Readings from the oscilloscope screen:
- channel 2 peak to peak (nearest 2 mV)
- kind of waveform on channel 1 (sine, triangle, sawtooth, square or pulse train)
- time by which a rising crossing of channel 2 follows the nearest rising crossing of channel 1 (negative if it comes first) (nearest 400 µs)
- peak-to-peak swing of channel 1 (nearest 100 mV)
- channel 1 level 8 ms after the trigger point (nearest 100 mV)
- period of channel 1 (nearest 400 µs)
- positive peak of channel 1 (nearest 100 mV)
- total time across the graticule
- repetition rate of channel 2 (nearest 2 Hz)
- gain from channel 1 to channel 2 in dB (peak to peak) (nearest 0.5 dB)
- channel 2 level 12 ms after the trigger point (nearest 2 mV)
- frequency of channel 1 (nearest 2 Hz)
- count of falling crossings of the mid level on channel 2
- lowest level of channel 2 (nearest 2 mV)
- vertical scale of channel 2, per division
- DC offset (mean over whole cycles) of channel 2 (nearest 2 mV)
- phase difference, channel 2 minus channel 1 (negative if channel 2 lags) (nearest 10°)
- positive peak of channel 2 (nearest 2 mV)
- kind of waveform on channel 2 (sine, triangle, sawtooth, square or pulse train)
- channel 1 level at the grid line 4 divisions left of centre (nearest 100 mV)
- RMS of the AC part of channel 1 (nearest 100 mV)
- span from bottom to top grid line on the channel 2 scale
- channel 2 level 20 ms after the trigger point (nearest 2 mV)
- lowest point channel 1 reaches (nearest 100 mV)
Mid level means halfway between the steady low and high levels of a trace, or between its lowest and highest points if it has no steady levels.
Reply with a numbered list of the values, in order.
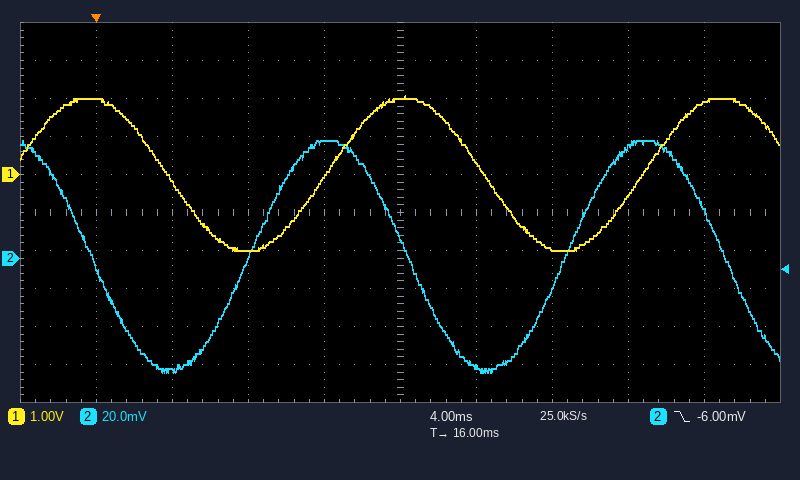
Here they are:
1. 122 mV
2. sine
3. -4.0 ms
4. 4.1 V
5. -2.0 V
6. 16.8 ms
7. 2.1 V
8. 40 ms
9. 60 Hz
10. -30.5 dB
11. 62 mV
12. 60 Hz
13. 3
14. -60 mV
15. 20 mV
16. 2 mV
17. +90°
18. 62 mV
19. sine
20. 2.0 V
21. 1.4 V
22. 200 mV
23. -58 mV
24. -2.0 V
